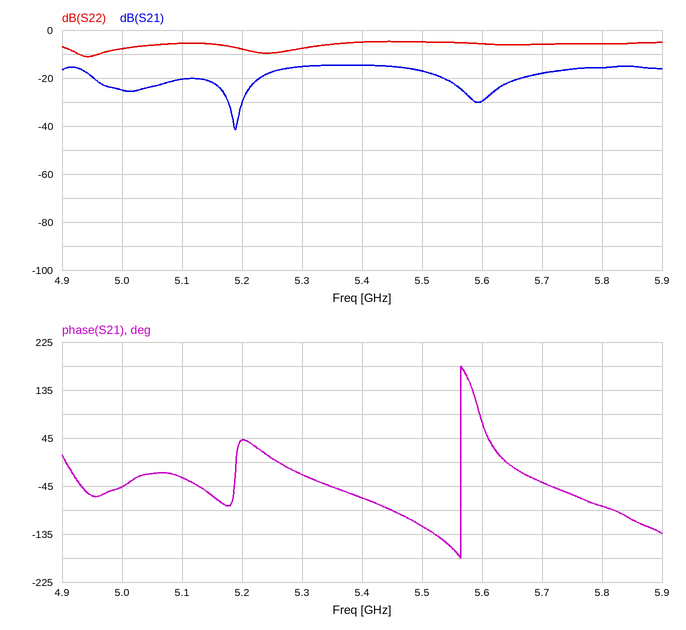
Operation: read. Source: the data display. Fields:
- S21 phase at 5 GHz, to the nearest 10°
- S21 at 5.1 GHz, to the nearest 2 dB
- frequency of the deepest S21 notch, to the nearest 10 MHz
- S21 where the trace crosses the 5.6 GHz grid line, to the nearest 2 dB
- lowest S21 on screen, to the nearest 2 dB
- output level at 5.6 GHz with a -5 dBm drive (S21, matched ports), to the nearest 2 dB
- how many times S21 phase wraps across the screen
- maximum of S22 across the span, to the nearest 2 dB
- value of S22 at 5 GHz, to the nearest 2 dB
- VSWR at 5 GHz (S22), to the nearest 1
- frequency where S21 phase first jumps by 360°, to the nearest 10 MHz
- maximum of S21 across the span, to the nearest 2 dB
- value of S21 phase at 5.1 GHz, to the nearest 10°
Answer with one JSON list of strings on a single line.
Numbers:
["-50°", "-20 dB", "5.19 GHz", "-30 dB", "-42 dB", "-34 dBm", "1", "-4 dB", "-8 dB", "2", "5.56 GHz", "-14 dB", "-30°"]
